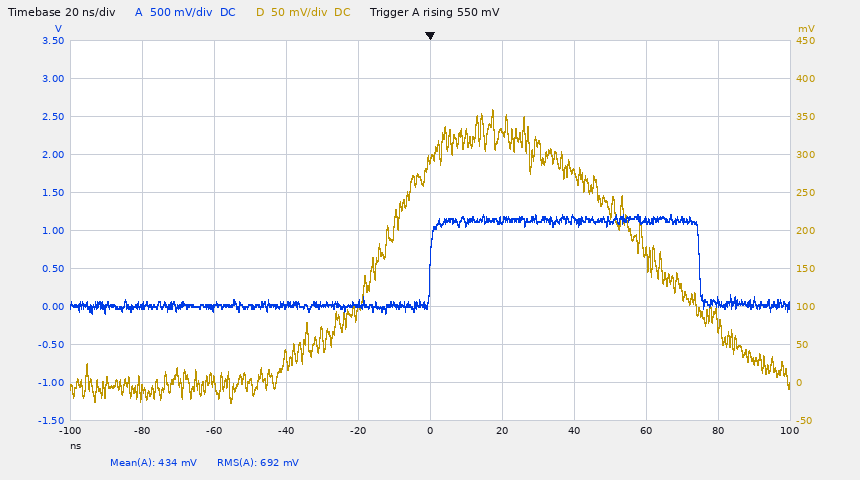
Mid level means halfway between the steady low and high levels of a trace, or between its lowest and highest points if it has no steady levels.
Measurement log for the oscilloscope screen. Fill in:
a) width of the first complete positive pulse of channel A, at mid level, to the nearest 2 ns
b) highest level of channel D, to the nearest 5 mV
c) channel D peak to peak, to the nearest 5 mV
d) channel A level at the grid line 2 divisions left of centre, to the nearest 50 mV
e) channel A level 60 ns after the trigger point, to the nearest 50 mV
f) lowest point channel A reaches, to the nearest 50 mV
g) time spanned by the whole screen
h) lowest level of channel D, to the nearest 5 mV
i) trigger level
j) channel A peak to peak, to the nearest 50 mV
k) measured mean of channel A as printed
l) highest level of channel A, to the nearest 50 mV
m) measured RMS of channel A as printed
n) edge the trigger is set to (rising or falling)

74 ns
360 mV
385 mV
0 mV
1.15 V
-100 mV
200 ns
-25 mV
550 mV
1.30 V
434 mV
1.20 V
692 mV
rising
